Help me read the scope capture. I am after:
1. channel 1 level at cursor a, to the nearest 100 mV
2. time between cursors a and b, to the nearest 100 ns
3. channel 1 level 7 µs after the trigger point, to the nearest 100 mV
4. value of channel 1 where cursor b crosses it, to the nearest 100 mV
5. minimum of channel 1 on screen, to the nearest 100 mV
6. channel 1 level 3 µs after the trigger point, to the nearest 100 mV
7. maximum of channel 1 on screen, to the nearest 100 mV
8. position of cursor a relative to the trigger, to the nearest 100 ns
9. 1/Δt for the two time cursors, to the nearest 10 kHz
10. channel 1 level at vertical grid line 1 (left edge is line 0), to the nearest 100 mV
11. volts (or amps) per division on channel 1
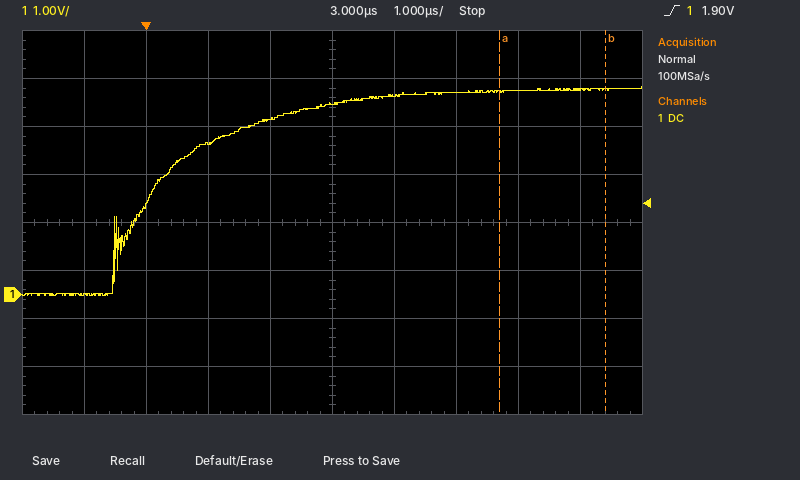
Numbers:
4.2 V
1.7 µs
4.3 V
4.3 V
0.0 V
4.0 V
4.3 V
+5.7 µs
590 kHz
0.0 V
1 V
